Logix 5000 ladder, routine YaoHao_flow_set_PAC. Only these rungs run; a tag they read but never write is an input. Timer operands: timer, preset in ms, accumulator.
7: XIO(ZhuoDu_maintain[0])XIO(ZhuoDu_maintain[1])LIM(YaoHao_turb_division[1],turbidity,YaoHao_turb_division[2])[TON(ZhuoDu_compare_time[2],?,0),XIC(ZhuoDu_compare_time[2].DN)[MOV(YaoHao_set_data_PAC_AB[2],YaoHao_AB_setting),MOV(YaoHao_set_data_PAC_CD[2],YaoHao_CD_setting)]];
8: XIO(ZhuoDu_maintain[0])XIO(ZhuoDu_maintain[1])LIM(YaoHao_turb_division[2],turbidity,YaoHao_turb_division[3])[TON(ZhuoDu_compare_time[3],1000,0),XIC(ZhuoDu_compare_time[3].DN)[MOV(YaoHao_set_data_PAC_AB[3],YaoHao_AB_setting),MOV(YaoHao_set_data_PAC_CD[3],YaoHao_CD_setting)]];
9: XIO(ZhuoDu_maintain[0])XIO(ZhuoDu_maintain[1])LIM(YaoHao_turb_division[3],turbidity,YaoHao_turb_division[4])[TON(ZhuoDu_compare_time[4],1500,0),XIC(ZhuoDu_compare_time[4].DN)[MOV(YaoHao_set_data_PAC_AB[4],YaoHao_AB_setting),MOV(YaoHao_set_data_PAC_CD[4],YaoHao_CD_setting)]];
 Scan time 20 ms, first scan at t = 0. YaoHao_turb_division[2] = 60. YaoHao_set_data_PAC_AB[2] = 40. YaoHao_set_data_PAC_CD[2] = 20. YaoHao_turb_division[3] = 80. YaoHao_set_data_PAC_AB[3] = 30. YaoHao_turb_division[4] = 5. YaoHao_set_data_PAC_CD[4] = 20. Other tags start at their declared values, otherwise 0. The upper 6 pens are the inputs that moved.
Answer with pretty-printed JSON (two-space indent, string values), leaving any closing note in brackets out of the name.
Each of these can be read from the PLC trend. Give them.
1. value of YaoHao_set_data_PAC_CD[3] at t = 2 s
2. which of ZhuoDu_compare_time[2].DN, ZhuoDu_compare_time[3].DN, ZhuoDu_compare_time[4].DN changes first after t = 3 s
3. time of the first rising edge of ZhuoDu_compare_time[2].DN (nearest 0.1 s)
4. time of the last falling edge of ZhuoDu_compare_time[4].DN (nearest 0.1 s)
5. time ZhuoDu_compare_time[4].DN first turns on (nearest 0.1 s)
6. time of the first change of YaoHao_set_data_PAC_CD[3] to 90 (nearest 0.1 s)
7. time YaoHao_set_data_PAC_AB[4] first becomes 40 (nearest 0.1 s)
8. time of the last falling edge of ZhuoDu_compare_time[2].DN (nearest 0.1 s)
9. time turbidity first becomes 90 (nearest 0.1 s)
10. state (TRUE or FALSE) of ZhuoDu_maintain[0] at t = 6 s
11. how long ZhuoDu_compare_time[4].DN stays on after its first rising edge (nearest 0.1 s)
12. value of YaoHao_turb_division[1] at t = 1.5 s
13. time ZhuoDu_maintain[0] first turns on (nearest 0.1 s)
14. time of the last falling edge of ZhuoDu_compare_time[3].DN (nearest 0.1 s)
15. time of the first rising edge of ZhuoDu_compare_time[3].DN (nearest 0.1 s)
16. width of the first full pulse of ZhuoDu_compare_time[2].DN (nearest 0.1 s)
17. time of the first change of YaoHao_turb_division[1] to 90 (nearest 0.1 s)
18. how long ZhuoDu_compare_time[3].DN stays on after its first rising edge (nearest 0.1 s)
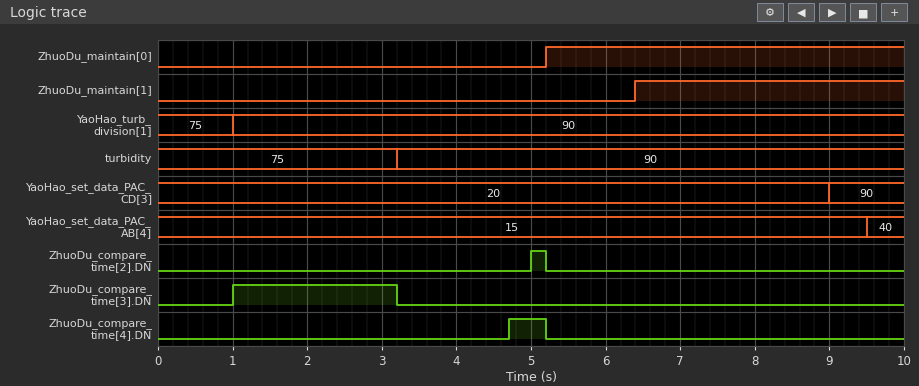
{
  "value of YaoHao_set_data_PAC_CD[3] at t = 2 s": "20",
  "which of ZhuoDu_compare_time[2].DN, ZhuoDu_compare_time[3].DN, ZhuoDu_compare_time[4].DN changes first after t = 3 s": "ZhuoDu_compare_time[3].DN",
  "time of the first rising edge of ZhuoDu_compare_time[2].DN": "5.0 s",
  "time of the last falling edge of ZhuoDu_compare_time[4].DN": "5.2 s",
  "time ZhuoDu_compare_time[4].DN first turns on": "4.7 s",
  "time of the first change of YaoHao_set_data_PAC_CD[3] to 90": "9.0 s",
  "time YaoHao_set_data_PAC_AB[4] first becomes 40": "9.5 s",
  "time of the last falling edge of ZhuoDu_compare_time[2].DN": "5.2 s",
  "time turbidity first becomes 90": "3.2 s",
  "state (TRUE or FALSE) of ZhuoDu_maintain[0] at t = 6 s": "TRUE",
  "how long ZhuoDu_compare_time[4].DN stays on after its first rising edge": "0.5 s",
  "value of YaoHao_turb_division[1] at t = 1.5 s": "90",
  "time ZhuoDu_maintain[0] first turns on": "5.2 s",
  "time of the last falling edge of ZhuoDu_compare_time[3].DN": "3.2 s",
  "time of the first rising edge of ZhuoDu_compare_time[3].DN": "1.0 s",
  "width of the first full pulse of ZhuoDu_compare_time[2].DN": "0.2 s",
  "time of the first change of YaoHao_turb_division[1] to 90": "1.0 s",
  "how long ZhuoDu_compare_time[3].DN stays on after its first rising edge": "2.2 s"
}
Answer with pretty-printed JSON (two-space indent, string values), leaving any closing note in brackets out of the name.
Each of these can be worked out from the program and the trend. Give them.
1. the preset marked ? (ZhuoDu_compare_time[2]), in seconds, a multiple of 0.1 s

{
  "the preset marked ? (ZhuoDu_compare_time[2]), in seconds, a multiple of 0.1 s": "1.8 s"
}
